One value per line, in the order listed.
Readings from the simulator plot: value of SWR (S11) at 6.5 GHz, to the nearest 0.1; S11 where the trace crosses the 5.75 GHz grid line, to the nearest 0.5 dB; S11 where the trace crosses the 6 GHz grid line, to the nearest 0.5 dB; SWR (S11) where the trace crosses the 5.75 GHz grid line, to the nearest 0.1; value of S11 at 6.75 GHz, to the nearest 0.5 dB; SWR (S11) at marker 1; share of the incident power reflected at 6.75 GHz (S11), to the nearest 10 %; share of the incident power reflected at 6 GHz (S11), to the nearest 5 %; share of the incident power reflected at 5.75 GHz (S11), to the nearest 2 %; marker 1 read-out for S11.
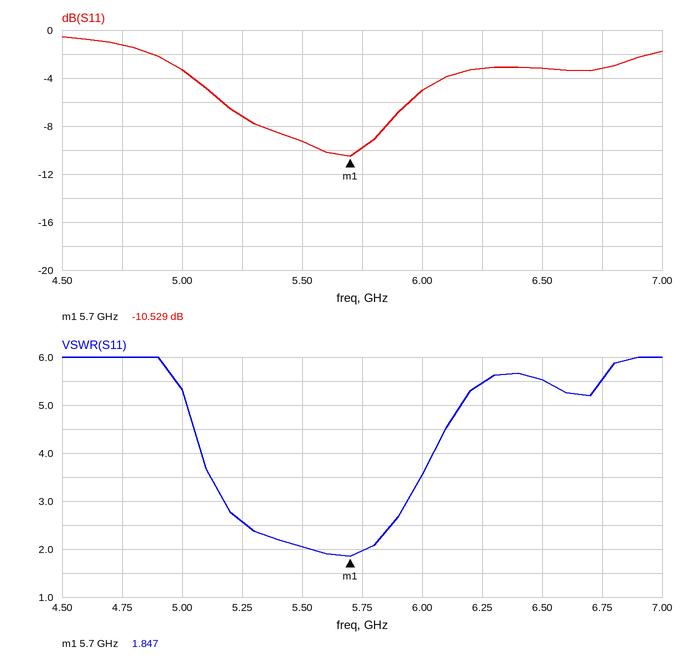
5.5
-10.0 dB
-5.0 dB
2.0
-3.0 dB
1.847
50 %
30 %
10 %
-10.529 dB
